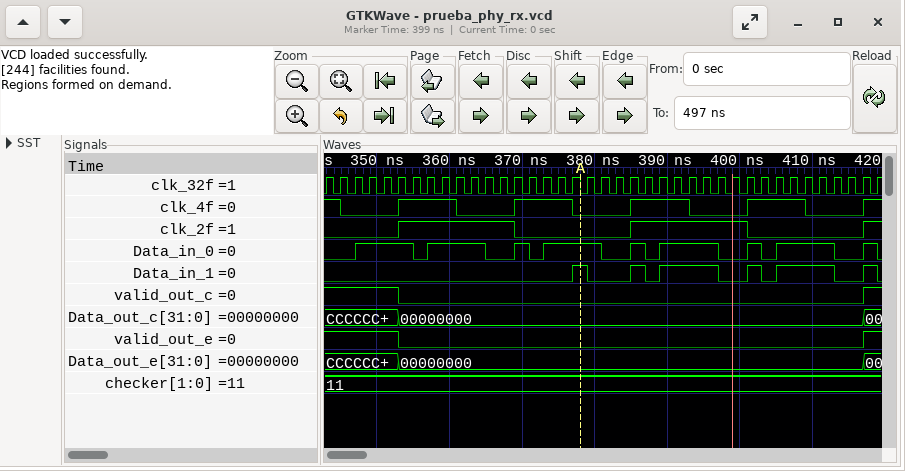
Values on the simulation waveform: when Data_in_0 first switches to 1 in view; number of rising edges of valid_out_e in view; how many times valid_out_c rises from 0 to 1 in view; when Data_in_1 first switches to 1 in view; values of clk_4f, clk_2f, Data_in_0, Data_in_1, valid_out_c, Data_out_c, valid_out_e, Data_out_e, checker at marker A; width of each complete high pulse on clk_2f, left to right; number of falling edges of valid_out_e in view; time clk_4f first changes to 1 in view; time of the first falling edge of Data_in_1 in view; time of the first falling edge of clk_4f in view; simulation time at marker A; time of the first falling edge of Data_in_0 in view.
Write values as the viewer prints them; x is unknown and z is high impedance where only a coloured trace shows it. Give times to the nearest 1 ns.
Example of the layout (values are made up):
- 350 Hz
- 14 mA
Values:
- 347 ns
- 1
- 1
- 377 ns
- clk_4f=0, clk_2f=0, Data_in_0=1, Data_in_1=1, valid_out_c=0, Data_out_c=00000000, valid_out_e=0, Data_out_e=00000000, checker=11
- 16 ns, 16 ns
- 1
- 353 ns
- 379 ns
- 345 ns
- 378 ns
- 355 ns
